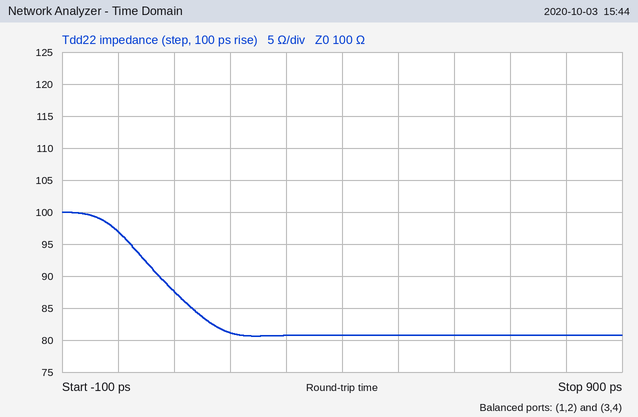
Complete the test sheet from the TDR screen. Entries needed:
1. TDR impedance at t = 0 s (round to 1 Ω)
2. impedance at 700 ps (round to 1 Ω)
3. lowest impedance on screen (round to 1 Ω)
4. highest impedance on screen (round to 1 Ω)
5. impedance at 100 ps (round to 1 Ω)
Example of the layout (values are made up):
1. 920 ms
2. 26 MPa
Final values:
1. 97 Ω
2. 81 Ω
3. 81 Ω
4. 100 Ω
5. 88 Ω
